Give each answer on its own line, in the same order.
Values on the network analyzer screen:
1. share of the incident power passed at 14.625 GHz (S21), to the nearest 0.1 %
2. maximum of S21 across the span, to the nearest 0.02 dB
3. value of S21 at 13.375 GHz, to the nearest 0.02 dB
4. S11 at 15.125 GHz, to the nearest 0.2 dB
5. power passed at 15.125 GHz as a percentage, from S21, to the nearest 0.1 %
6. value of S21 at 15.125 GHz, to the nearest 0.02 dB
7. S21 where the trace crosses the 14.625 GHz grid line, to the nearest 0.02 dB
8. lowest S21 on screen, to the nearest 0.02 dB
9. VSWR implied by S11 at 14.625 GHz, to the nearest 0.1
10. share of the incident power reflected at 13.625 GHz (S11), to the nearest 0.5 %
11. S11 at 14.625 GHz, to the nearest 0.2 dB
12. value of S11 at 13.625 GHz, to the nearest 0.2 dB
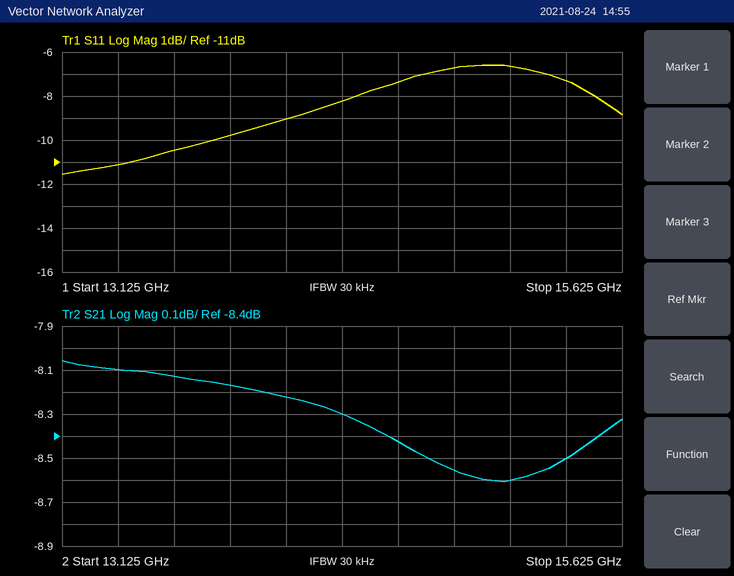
14.4 %
-8.06 dB
-8.10 dB
-6.6 dB
13.8 %
-8.60 dB
-8.42 dB
-8.60 dB
2.5
9.0 %
-7.4 dB
-10.4 dB
